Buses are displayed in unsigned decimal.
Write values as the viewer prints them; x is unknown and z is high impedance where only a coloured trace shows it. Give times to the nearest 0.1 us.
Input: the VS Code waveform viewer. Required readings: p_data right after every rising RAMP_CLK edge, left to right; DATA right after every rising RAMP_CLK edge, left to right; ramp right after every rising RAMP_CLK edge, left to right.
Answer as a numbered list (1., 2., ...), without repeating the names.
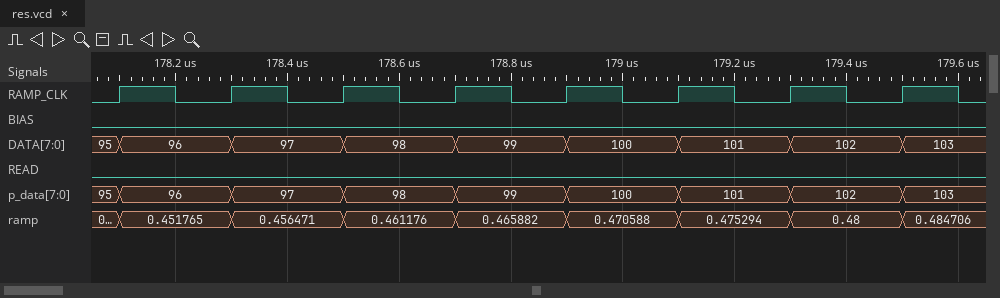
1. 96, 97, 98, 99, 100, 101, 102, 103
2. 96, 97, 98, 99, 100, 101, 102, 103
3. 0.451765, 0.456471, 0.461176, 0.465882, 0.470588, 0.475294, 0.48, 0.484706
